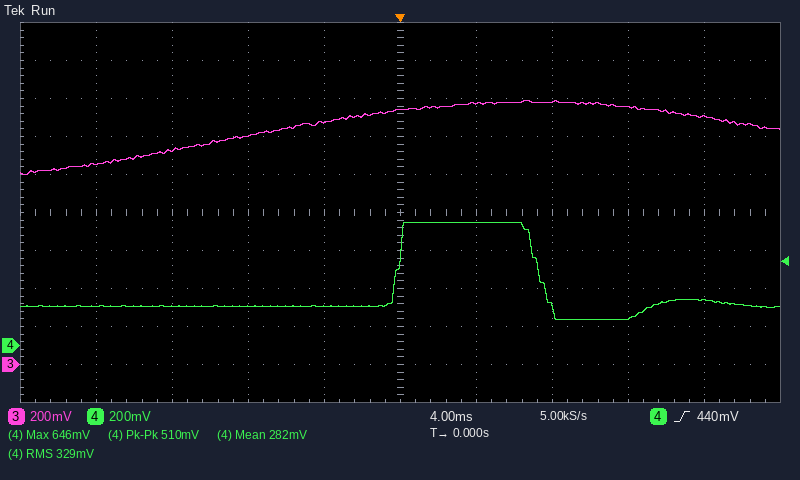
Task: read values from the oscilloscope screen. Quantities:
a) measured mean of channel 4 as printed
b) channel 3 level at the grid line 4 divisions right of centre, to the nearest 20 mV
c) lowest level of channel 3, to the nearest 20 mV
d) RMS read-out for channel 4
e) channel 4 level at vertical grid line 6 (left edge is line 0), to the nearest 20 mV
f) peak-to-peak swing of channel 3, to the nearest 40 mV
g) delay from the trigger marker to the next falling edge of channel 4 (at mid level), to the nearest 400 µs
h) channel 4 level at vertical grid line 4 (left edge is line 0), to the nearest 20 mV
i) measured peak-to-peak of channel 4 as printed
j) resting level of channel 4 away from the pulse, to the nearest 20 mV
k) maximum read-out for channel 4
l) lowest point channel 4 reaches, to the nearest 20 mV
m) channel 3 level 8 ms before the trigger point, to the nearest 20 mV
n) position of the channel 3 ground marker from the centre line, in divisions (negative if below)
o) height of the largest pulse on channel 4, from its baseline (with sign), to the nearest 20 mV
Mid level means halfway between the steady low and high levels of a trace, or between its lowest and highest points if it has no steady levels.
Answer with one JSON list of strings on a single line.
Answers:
["282 mV", "1.30 V", "1.00 V", "329 mV", "640 mV", "400 mV", "7.2 ms", "200 mV", "510 mV", "200 mV", "646 mV", "140 mV", "1.20 V", "-4.0 div", "+440 mV"]
